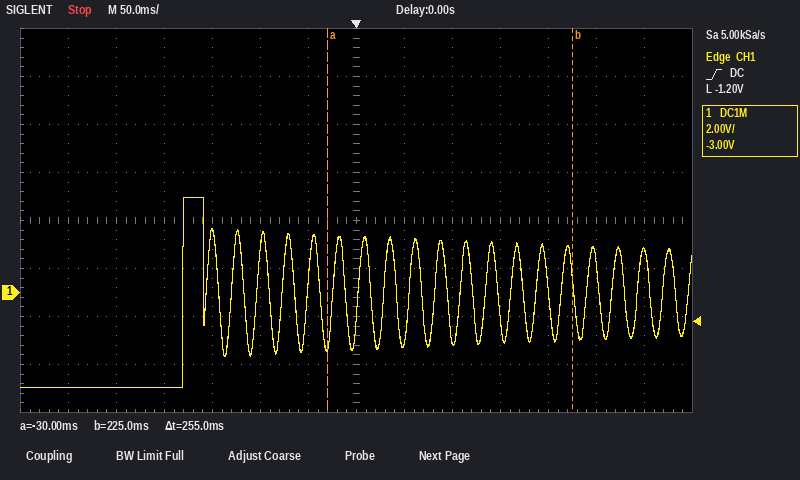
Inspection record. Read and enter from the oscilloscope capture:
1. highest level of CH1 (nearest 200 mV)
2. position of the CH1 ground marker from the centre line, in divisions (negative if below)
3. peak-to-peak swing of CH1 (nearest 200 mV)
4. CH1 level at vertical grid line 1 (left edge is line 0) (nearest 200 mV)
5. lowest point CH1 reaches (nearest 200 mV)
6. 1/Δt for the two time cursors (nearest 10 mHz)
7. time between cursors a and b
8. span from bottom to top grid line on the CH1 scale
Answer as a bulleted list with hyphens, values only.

- 4.0 V
- -1.5 div
- 8.0 V
- -4.0 V
- -4.0 V
- 3.92 Hz
- 255 ms
- 16 V
